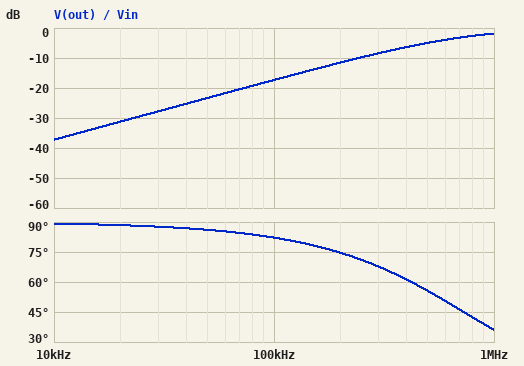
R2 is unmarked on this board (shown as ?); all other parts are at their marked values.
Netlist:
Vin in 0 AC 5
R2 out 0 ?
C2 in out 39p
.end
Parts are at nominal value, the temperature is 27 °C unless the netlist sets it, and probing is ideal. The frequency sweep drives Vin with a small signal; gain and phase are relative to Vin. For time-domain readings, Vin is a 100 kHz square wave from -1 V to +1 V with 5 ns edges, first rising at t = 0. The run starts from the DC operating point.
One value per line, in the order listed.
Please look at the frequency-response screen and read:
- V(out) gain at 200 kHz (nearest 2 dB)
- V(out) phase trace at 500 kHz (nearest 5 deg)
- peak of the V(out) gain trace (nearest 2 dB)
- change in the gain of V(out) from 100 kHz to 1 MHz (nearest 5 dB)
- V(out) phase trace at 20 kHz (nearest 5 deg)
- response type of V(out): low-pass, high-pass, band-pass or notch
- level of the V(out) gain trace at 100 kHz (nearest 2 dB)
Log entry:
-12 dB
55 deg
-2 dB
15 dB
90 deg
high-pass
-18 dB
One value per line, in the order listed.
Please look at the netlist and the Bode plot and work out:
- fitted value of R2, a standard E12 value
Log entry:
5.6 kΩ
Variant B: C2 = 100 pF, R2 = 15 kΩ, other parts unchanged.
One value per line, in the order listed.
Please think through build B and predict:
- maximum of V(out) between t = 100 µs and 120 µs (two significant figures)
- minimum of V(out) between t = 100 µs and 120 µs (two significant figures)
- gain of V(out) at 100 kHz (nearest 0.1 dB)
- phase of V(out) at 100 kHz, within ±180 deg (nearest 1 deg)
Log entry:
1.9 V
-1.9 V
-3.3 dB
47 deg
